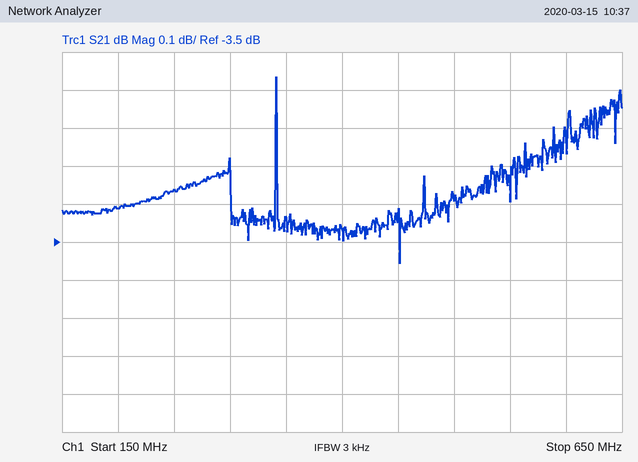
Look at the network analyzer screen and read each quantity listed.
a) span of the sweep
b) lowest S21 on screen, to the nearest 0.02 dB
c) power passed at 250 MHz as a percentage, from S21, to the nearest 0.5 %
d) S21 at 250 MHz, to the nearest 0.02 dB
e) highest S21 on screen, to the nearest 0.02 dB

500 MHz
-3.56 dB
46.0 %
-3.36 dB
-3.06 dB
